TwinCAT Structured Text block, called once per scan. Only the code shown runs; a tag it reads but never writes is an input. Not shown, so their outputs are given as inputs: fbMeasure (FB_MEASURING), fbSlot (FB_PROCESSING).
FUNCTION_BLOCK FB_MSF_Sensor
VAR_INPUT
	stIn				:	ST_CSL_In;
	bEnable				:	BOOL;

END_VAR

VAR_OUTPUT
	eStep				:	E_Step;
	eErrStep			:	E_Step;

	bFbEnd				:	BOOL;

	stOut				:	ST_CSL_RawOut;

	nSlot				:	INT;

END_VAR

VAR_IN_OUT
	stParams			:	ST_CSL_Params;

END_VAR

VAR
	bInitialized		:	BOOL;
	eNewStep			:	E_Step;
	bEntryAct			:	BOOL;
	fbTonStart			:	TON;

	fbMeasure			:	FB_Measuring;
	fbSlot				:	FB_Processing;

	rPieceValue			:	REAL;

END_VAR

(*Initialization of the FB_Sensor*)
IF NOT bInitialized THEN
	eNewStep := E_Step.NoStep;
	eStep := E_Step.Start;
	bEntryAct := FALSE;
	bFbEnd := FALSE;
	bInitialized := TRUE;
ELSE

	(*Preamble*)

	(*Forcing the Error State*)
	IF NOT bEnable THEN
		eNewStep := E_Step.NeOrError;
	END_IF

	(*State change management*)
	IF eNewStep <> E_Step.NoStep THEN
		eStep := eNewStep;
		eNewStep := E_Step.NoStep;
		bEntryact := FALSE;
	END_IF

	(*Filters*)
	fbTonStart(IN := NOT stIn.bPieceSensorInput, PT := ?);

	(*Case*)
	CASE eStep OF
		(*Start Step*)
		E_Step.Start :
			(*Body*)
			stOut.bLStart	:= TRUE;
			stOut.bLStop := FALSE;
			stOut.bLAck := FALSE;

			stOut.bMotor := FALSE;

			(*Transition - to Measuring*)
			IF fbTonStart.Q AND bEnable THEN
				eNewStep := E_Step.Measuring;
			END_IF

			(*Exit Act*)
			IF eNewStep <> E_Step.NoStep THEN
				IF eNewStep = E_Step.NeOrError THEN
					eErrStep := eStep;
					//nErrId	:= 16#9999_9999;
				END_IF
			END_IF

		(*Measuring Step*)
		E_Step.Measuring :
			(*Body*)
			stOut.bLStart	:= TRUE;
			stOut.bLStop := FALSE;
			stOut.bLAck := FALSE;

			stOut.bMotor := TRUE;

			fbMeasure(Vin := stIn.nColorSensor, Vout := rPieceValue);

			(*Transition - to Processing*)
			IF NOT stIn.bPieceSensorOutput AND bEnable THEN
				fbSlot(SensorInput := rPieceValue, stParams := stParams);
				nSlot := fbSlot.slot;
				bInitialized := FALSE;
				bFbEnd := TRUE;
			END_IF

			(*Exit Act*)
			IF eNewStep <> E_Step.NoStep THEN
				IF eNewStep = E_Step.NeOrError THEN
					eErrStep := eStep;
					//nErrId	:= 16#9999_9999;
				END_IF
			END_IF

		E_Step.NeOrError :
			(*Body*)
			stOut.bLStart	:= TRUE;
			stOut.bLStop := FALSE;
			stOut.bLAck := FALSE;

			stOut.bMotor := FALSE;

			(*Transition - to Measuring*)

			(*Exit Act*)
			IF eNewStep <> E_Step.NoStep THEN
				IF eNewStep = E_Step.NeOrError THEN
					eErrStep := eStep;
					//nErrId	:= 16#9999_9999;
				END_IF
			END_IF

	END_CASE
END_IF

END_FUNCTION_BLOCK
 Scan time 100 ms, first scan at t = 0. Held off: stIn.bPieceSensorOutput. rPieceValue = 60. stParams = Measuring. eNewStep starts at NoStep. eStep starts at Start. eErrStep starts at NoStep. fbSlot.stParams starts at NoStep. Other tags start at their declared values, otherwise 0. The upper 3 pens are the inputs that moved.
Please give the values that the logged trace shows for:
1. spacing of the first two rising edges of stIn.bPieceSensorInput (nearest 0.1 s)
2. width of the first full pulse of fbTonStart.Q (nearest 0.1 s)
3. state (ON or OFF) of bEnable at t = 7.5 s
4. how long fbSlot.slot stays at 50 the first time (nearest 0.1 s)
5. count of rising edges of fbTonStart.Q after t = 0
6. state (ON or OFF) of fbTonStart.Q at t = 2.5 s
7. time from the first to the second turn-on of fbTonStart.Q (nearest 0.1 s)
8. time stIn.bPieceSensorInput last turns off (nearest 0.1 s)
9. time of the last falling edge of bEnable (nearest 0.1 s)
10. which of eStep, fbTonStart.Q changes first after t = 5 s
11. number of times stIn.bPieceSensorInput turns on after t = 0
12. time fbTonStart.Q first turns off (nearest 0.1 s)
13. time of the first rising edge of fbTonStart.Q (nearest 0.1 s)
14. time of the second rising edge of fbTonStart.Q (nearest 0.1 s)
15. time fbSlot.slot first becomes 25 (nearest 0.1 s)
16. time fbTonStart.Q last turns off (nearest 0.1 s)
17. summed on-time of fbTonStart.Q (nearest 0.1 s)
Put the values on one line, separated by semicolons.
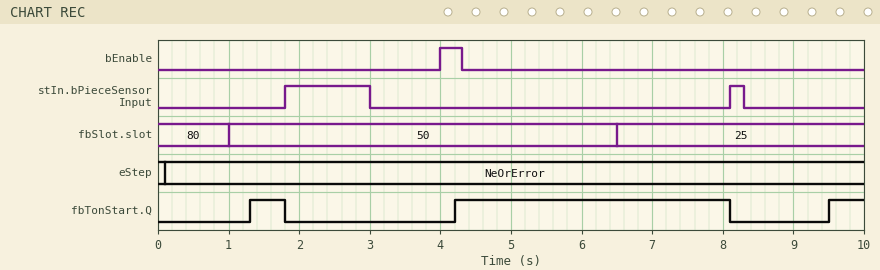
6.3 s; 0.5 s; OFF; 5.5 s; 3; OFF; 2.9 s; 8.3 s; 4.3 s; fbTonStart.Q; 2; 1.8 s; 1.3 s; 4.2 s; 6.5 s; 8.1 s; 4.9 s
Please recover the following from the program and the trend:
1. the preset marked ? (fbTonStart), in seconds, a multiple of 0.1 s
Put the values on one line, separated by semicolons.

1.2 s
